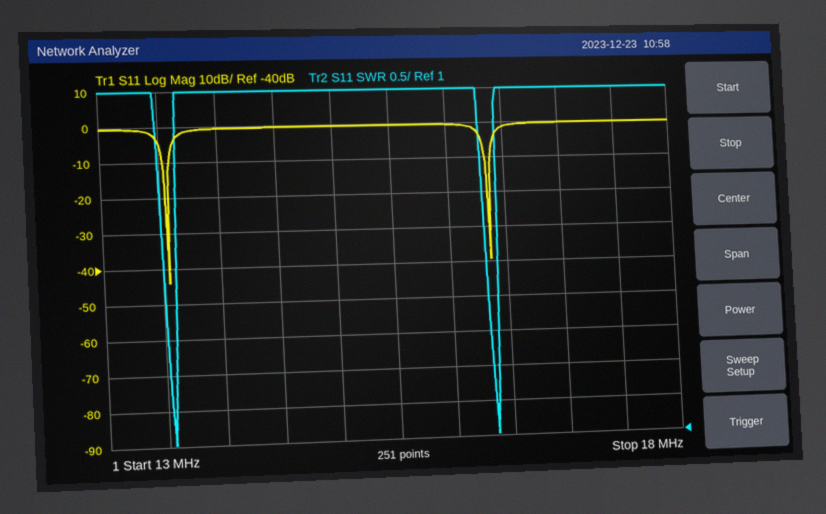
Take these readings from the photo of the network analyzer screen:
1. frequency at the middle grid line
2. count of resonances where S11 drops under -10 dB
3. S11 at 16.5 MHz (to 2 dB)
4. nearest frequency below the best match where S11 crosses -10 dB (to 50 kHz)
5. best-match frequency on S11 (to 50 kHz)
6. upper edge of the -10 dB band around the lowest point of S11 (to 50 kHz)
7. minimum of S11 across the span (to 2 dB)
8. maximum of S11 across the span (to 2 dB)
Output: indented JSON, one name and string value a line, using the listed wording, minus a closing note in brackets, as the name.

{
  "frequency at the middle grid line": "15.5 MHz",
  "count of resonances where S11 drops under -10 dB": "2",
  "S11 at 16.5 MHz": "-2 dB",
  "nearest frequency below the best match where S11 crosses -10 dB": "13.55 MHz",
  "best-match frequency on S11": "13.55 MHz",
  "upper edge of the -10 dB band around the lowest point of S11": "13.60 MHz",
  "minimum of S11 across the span": "-44 dB",
  "maximum of S11 across the span": "0 dB"
}
